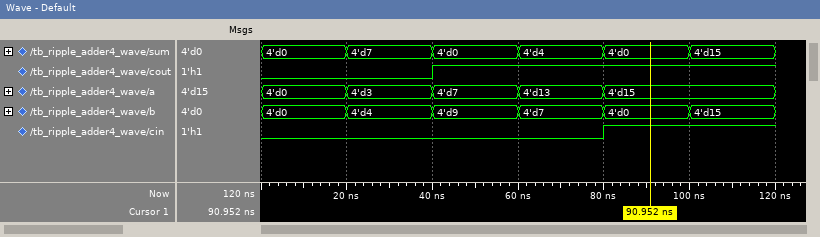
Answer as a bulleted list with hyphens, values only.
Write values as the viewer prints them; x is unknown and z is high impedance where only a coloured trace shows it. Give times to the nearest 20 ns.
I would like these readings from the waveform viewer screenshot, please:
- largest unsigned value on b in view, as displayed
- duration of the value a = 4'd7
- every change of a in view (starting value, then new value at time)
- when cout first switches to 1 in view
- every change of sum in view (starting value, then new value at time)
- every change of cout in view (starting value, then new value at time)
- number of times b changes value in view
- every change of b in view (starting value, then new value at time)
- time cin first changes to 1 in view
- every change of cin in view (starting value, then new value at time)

- 4'd15
- 20 ns
- 4'd0, 4'd3 at 20 ns, 4'd7 at 40 ns, 4'd13 at 60 ns, 4'd15 at 80 ns
- 40 ns
- 4'd0, 4'd7 at 20 ns, 4'd0 at 40 ns, 4'd4 at 60 ns, 4'd0 at 80 ns, 4'd15 at 100 ns
- 0, 1 at 40 ns
- 5
- 4'd0, 4'd4 at 20 ns, 4'd9 at 40 ns, 4'd7 at 60 ns, 4'd0 at 80 ns, 4'd15 at 100 ns
- 80 ns
- 0, 1 at 80 ns
